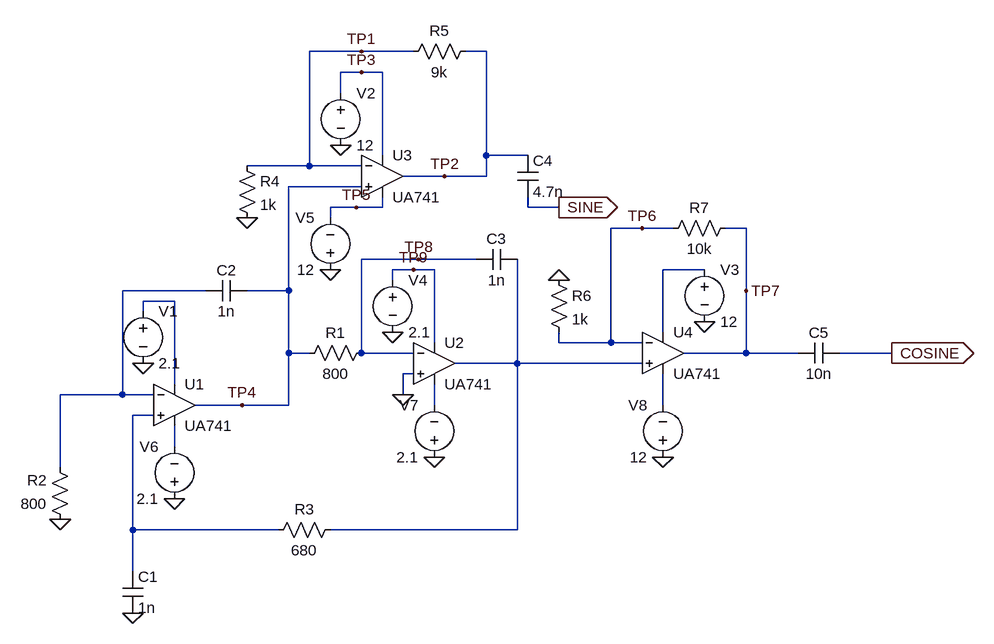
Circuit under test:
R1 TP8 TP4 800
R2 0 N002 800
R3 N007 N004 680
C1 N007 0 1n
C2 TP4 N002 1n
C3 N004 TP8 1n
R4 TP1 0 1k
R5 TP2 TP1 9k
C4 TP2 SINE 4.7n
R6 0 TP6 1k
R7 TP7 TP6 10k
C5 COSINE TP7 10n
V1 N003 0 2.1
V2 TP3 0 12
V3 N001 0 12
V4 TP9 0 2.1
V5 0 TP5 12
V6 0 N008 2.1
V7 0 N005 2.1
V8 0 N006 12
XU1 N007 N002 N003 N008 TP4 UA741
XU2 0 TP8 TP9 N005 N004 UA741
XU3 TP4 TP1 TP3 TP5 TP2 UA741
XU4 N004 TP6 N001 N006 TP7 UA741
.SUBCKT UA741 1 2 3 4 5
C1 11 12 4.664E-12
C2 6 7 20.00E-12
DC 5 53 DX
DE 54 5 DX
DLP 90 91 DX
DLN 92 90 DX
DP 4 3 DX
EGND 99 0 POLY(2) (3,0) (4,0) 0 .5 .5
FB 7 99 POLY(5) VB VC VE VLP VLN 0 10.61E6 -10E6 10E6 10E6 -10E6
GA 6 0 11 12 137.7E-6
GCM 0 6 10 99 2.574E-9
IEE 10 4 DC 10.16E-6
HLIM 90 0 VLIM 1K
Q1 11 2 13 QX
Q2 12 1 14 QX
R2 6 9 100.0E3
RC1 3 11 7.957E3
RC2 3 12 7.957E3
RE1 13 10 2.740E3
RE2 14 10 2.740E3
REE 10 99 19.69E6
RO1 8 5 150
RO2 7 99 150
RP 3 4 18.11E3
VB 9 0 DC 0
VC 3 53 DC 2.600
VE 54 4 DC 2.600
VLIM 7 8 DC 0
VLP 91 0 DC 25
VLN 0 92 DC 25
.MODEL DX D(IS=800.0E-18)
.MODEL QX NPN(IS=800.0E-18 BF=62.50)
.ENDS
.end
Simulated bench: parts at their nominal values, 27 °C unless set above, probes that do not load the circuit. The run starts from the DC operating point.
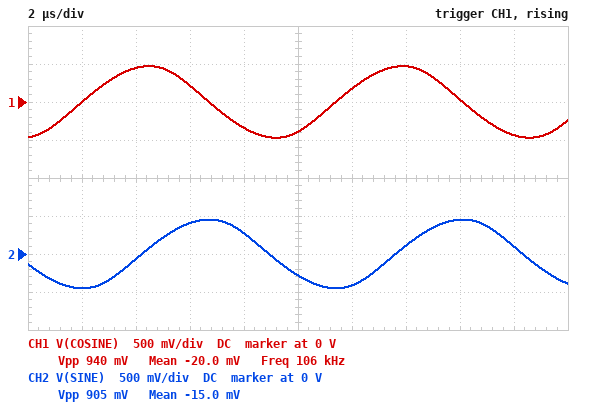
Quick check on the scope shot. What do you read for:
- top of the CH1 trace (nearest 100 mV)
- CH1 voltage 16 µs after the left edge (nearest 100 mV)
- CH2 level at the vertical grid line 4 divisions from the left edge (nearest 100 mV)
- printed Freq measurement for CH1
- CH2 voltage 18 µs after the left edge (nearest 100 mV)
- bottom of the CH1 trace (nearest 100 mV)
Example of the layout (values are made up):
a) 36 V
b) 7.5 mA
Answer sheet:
a) 500 mV
b) 0 V
c) 300 mV
d) 106 kHz
e) 100 mV
f) -500 mV
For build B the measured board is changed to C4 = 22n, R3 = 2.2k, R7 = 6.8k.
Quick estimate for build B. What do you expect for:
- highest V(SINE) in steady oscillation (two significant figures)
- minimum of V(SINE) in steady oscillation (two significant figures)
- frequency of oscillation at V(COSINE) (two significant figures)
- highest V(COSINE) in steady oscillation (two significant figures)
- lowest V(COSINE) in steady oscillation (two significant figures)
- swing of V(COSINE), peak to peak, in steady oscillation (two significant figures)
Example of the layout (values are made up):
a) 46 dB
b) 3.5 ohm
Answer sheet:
a) 670 mV
b) -670 mV
c) 72 kHz
d) 610 mV
e) -610 mV
f) 1.2 V
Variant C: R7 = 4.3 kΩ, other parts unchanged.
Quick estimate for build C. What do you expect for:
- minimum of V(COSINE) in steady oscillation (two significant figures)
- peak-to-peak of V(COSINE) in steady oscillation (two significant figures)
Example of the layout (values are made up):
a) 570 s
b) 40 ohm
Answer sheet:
a) -290 mV
b) 590 mV
